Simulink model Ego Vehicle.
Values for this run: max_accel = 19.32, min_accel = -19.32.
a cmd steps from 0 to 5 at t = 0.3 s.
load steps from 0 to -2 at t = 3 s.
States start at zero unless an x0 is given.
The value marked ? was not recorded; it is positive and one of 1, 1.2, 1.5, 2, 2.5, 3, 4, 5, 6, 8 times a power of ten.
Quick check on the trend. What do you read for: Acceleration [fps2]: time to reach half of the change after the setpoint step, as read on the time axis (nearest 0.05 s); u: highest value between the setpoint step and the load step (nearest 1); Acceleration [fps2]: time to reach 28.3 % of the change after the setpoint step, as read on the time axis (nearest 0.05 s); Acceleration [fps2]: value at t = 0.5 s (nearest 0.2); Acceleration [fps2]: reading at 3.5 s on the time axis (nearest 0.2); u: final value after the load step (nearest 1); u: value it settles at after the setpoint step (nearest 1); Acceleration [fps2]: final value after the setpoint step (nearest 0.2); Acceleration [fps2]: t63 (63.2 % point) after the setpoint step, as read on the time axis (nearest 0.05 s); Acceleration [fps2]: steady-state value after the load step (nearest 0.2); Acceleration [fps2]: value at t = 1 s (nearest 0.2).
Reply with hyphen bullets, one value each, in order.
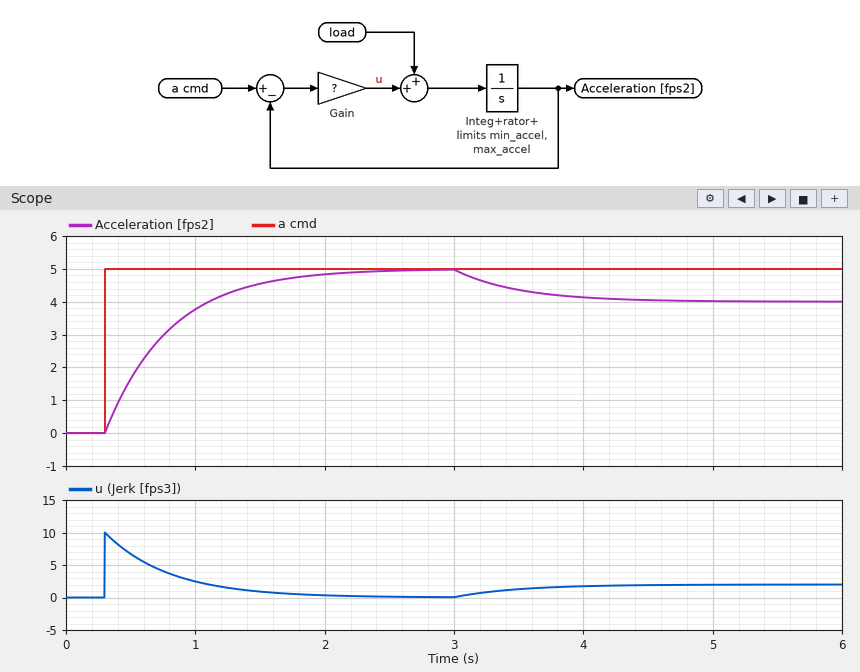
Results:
- 0.65 s
- 10
- 0.45 s
- 1.6
- 4.4
- 2
- 0
- 5.0
- 0.80 s
- 4.0
- 3.8
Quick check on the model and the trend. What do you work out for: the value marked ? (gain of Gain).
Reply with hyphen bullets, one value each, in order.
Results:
- 2
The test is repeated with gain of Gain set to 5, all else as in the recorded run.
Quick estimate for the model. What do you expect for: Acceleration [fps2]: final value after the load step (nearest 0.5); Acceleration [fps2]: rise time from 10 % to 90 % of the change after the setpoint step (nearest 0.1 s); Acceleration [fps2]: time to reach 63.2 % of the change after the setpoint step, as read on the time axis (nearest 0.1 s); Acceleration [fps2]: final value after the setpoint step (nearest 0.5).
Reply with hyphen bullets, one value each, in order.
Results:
- 4.5
- 0.4 s
- 0.5 s
- 5.0
